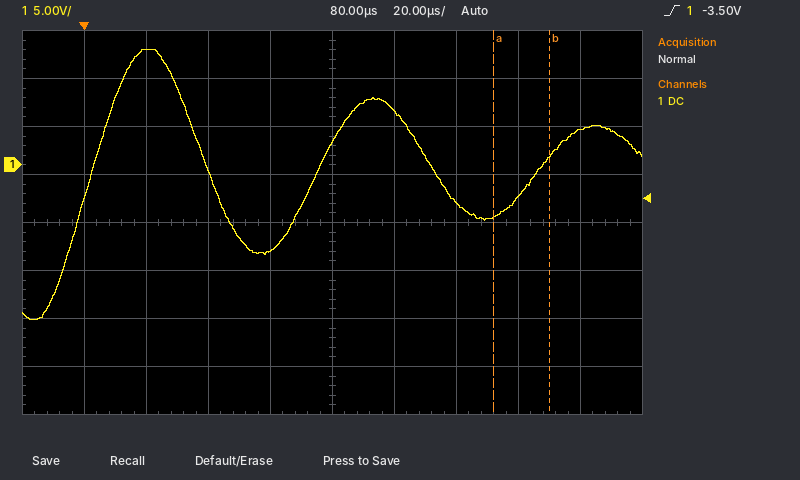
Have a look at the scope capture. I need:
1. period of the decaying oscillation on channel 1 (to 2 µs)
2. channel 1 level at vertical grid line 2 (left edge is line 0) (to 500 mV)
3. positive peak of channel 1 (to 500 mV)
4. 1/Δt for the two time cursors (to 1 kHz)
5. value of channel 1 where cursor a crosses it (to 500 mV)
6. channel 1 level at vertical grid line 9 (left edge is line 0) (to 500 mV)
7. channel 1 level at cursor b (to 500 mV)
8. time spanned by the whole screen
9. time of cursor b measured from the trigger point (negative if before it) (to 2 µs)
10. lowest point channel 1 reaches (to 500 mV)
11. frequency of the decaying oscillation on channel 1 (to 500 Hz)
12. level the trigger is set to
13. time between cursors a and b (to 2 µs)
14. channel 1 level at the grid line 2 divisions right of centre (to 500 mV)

72 µs
12.0 V
12.0 V
56 kHz
-5.5 V
3.5 V
1.0 V
200 µs
+150 µs
-16.0 V
14.0 kHz
-3.50 V
18 µs
-4.0 V
